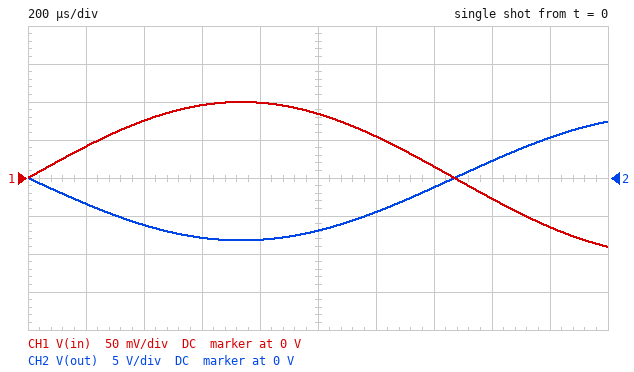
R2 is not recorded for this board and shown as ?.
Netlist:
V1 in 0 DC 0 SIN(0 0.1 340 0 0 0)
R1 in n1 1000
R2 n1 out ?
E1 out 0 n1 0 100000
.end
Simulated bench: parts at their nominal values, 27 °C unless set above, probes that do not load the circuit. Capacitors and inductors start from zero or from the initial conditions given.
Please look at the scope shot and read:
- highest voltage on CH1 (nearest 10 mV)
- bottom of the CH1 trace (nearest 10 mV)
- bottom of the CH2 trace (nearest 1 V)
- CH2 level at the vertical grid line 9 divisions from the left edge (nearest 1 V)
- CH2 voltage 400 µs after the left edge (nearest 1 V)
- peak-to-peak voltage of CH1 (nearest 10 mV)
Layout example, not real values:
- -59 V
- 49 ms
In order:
- 100 mV
- -90 mV
- -8 V
- 5 V
- -6 V
- 190 mV
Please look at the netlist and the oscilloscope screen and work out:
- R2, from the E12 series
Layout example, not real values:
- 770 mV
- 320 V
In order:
- 82 kΩ
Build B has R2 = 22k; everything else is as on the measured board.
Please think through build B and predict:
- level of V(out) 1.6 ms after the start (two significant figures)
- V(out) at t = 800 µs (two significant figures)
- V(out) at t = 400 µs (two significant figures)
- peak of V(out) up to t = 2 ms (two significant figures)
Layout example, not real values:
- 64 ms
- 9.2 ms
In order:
- 600 mV
- -2.2 V
- -1.7 V
- 2.0 V
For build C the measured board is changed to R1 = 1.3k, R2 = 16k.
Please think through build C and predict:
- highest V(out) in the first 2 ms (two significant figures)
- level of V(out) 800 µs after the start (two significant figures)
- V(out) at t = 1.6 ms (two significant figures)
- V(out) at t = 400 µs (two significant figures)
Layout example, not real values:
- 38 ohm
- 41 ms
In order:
- 1.1 V
- -1.2 V
- 340 mV
- -930 mV
